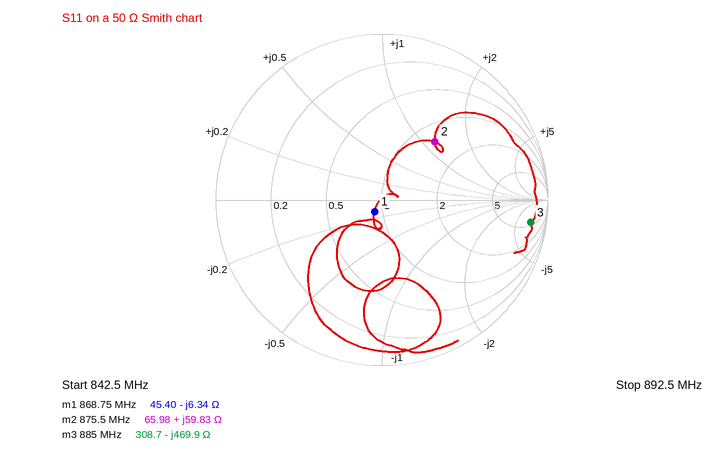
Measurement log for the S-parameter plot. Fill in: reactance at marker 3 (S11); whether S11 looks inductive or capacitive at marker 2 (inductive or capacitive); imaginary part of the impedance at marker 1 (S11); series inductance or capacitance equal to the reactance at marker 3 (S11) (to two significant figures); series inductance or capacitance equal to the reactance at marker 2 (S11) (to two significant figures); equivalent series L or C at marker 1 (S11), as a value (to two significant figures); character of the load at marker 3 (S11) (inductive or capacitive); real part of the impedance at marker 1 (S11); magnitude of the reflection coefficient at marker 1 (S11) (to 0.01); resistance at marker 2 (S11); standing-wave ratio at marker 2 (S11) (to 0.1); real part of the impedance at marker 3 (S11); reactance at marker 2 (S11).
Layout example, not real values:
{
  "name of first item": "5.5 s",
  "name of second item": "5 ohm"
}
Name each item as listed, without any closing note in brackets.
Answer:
{
  "reactance at marker 3": "-469.9 Ω",
  "whether S11 looks inductive or capacitive at marker 2": "inductive",
  "imaginary part of the impedance at marker 1": "-6.34 Ω",
  "series inductance or capacitance equal to the reactance at marker 3 (S11)": "380 fF",
  "series inductance or capacitance equal to the reactance at marker 2 (S11)": "11 nH",
  "equivalent series L or C at marker 1 (S11), as a value": "29 pF",
  "character of the load at marker 3 (S11)": "capacitive",
  "real part of the impedance at marker 1": "45.40 Ω",
  "magnitude of the reflection coefficient at marker 1 (S11)": "0.08",
  "resistance at marker 2": "65.98 Ω",
  "standing-wave ratio at marker 2 (S11)": "2.8",
  "real part of the impedance at marker 3": "308.7 Ω",
  "reactance at marker 2": "+59.83 Ω"
}
